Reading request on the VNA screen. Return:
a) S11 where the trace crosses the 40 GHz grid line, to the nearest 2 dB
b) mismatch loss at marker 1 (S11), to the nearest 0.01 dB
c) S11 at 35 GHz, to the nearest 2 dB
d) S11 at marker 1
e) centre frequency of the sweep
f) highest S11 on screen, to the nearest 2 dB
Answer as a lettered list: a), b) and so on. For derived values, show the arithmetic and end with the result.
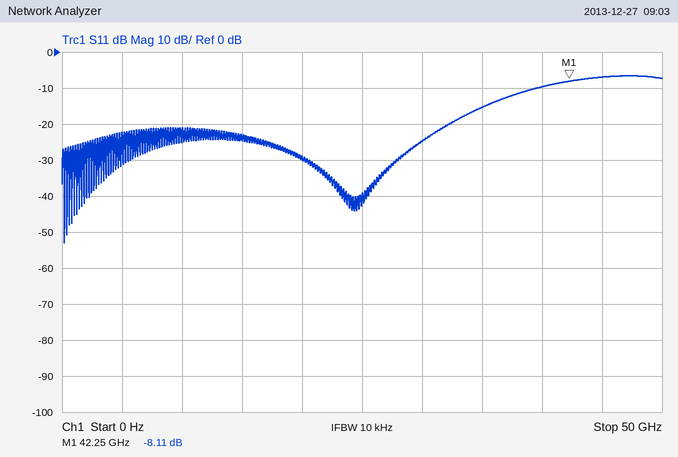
a) -10 dB
b) −10 log10(1 − 10^(-8.11/10)) ≈ 0.73 dB
c) -16 dB
d) -8.11 dB
e) 25 GHz
f) -6 dB
